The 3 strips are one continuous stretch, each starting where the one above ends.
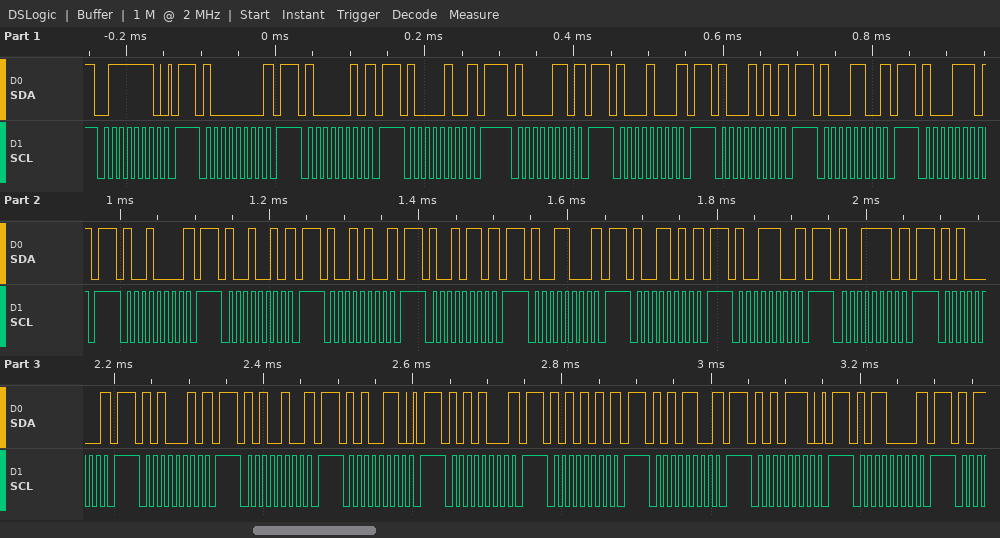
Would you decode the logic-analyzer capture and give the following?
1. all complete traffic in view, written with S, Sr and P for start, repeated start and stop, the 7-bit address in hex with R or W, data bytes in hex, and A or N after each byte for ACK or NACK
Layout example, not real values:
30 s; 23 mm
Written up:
S 3FW A P S 40W N P S 41W N P S 42W N P S 43W N P S 44W N P S 45W N P S 46W N P S 47W N P S 48W N P S 49W N P S 4AW N P S 4BW N P S 4CW N P S 4DW N P S 4EW N P S 4FW N P S 50W N P S 51W N P S 52W N P S 53W A P S 54W N P S 55W N P S 56W N P S 57W A P S 58W N P
